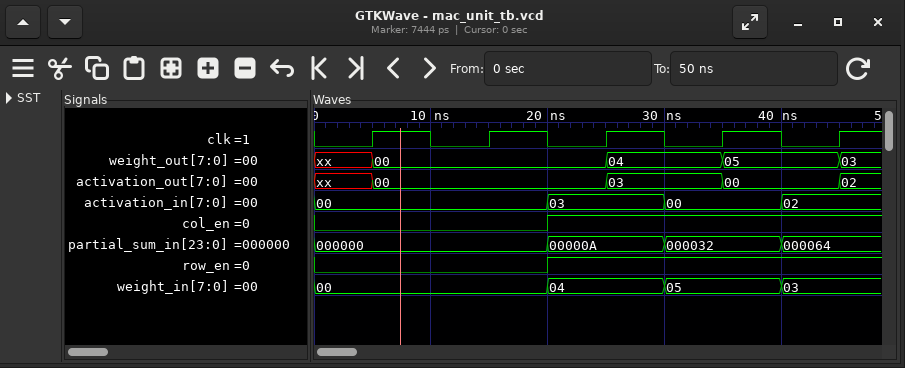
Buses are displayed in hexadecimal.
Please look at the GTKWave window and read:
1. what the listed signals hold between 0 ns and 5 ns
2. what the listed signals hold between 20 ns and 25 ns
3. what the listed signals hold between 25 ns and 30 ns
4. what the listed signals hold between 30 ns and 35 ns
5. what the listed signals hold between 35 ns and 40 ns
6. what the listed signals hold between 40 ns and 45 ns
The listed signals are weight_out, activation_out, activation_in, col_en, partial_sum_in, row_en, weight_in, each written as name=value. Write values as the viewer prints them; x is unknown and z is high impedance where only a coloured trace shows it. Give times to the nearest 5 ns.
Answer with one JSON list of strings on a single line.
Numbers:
["weight_out=xx, activation_out=xx, activation_in=00, col_en=0, partial_sum_in=000000, row_en=0, weight_in=00", "weight_out=00, activation_out=00, activation_in=03, col_en=1, partial_sum_in=00000A, row_en=1, weight_in=04", "weight_out=04, activation_out=03, activation_in=03, col_en=1, partial_sum_in=00000A, row_en=1, weight_in=04", "weight_out=04, activation_out=03, activation_in=00, col_en=1, partial_sum_in=000032, row_en=1, weight_in=05", "weight_out=05, activation_out=00, activation_in=00, col_en=1, partial_sum_in=000032, row_en=1, weight_in=05", "weight_out=05, activation_out=00, activation_in=02, col_en=1, partial_sum_in=000064, row_en=1, weight_in=03"]
